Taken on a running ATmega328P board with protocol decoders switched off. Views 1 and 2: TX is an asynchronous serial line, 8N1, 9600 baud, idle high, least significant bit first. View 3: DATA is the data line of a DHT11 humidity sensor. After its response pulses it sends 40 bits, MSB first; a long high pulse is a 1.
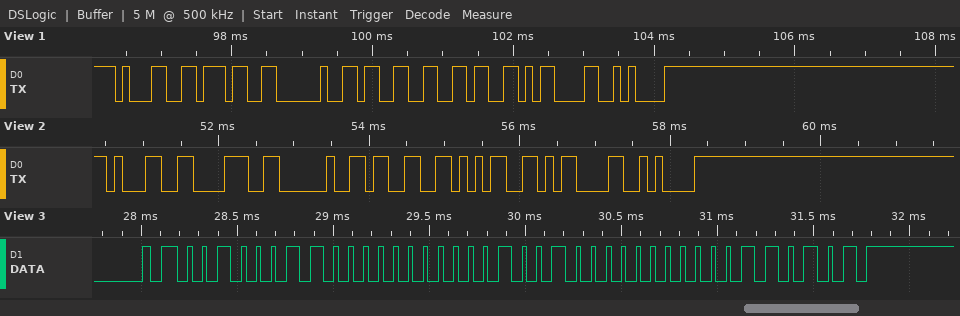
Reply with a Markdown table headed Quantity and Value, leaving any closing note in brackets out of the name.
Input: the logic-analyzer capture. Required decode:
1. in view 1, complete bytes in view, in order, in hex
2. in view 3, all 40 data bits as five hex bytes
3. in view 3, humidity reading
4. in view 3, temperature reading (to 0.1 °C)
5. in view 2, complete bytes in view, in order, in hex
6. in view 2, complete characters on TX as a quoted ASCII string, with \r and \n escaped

| Quantity | Value |
|---|---|
| in view 1, complete bytes in view, in order, in hex | 31 37 20 33 36 0D 0A |
| in view 3, all 40 data bits as five hex bytes | 23 00 12 00 35 |
| in view 3, humidity reading | 35 % |
| in view 3, temperature reading | 18.0 °C |
| in view 2, complete bytes in view, in order, in hex | 31 38 20 33 35 0D 0A |
| in view 2, complete characters on TX as a quoted ASCII string, with \r and \n escaped | "18 35\r\n" |
